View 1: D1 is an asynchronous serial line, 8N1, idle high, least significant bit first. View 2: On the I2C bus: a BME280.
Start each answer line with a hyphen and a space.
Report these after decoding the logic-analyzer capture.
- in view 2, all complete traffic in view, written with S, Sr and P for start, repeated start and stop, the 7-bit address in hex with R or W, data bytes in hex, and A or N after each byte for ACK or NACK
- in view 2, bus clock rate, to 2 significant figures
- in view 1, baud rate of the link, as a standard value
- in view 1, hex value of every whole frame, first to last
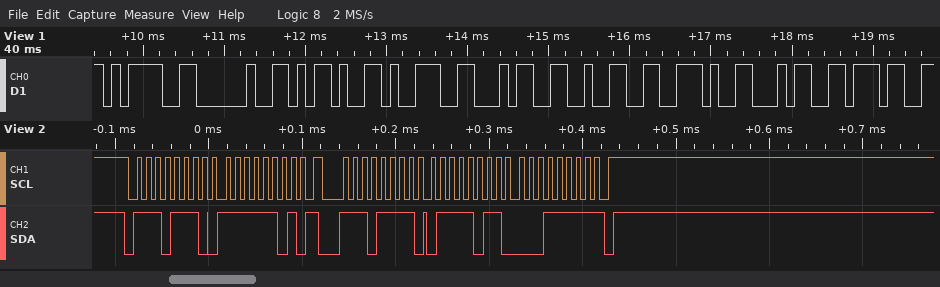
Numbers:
- S 77W A FD A Sr 77R A 7B A 1F N P
- 100 kHz
- 9600 baud
- 0x3D 0x20 0x2D 0x39 0x34 0x32 0x2E 0x34 0x37
